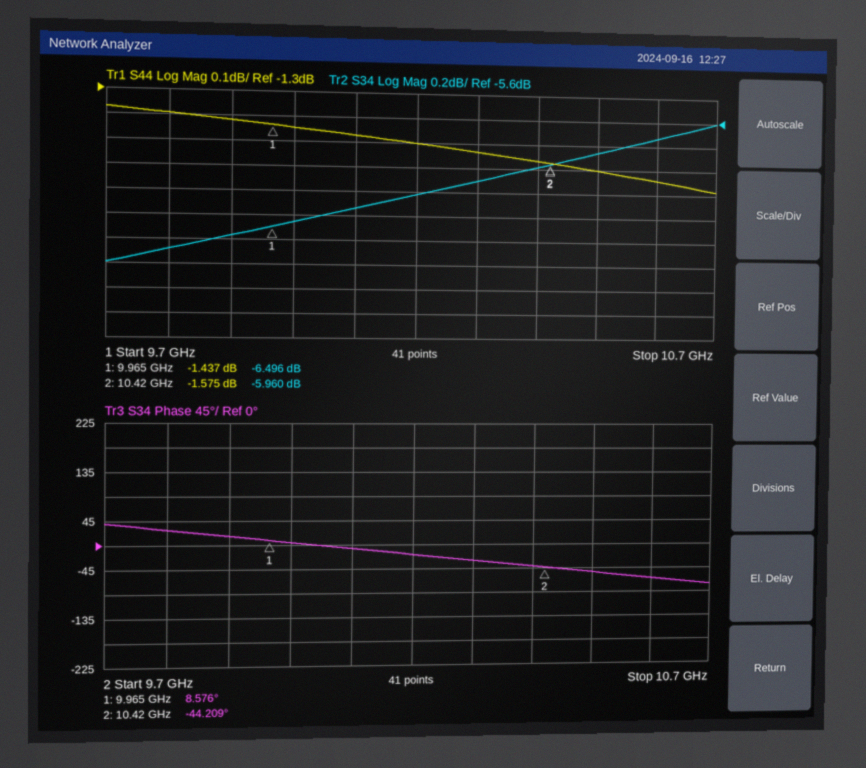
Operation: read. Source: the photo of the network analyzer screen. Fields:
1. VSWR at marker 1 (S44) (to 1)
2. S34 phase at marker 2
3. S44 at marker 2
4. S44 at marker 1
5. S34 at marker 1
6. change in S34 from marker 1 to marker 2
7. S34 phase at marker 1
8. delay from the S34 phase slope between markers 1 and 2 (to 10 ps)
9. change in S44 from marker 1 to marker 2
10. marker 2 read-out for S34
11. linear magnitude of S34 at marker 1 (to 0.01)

12
-44.209°
-1.575 dB
-1.437 dB
-6.496 dB
0.536 dB
8.576°
320 ps
-0.138 dB
-5.960 dB
0.47
